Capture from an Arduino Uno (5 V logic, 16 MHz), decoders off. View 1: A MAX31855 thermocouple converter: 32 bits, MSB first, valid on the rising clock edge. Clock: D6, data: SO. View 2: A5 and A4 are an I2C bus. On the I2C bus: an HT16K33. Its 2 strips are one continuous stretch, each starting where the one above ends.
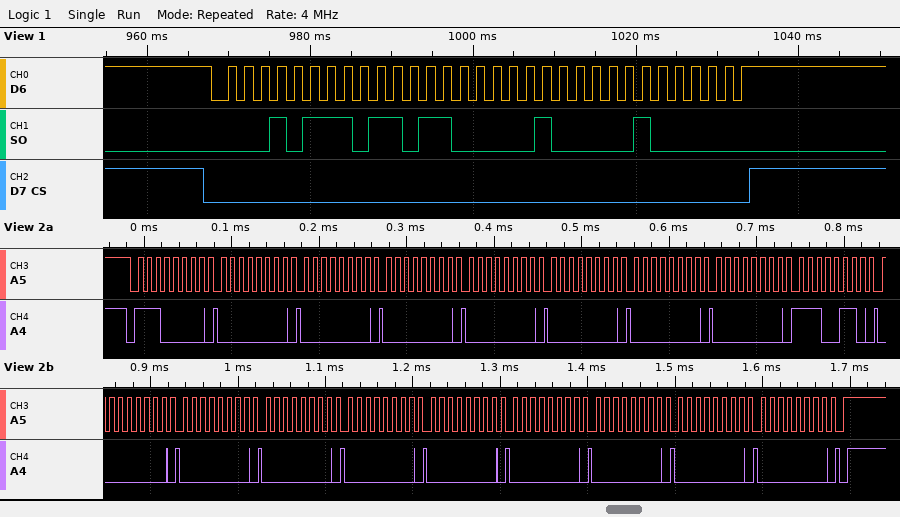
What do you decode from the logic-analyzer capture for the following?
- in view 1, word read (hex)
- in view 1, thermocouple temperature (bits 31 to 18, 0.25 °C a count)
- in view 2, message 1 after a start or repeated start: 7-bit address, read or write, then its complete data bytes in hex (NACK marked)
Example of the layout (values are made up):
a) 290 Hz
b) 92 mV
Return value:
a) 0x176C1040
b) 374.75 °C
c) 0x70 write: 00 00 00 00 00 00 00 E6 00 00 00 00 00 00 00 00 00
